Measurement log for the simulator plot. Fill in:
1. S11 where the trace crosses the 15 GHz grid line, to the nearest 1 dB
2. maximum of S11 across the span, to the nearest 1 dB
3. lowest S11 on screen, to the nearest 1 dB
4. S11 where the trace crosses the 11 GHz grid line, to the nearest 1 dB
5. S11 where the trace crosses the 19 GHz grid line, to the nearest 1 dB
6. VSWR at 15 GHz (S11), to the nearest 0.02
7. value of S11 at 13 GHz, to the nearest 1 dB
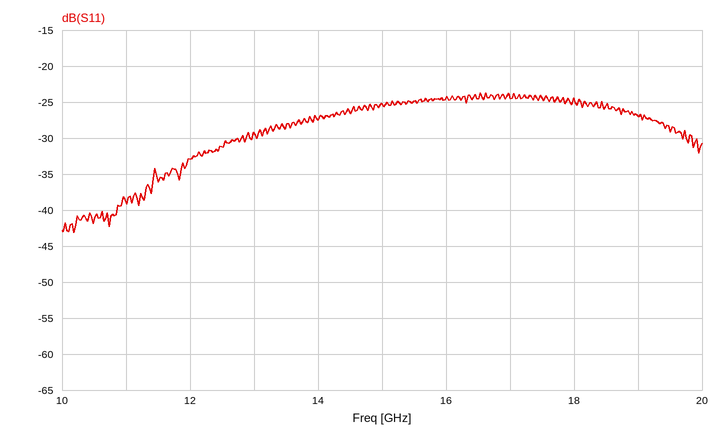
-25 dB
-24 dB
-43 dB
-39 dB
-27 dB
1.12
-29 dB
